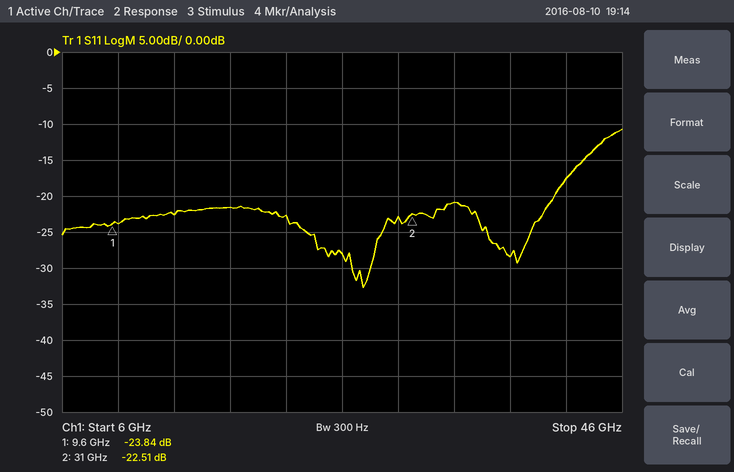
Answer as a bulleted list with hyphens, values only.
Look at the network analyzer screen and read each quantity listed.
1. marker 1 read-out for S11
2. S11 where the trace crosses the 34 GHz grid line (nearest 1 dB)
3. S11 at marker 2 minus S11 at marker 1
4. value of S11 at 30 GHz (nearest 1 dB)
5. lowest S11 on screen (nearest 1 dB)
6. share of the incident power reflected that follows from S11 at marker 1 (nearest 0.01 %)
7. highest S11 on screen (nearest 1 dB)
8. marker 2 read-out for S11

- -23.84 dB
- -21 dB
- 1.33 dB
- -23 dB
- -33 dB
- 0.41 %
- -11 dB
- -22.51 dB
